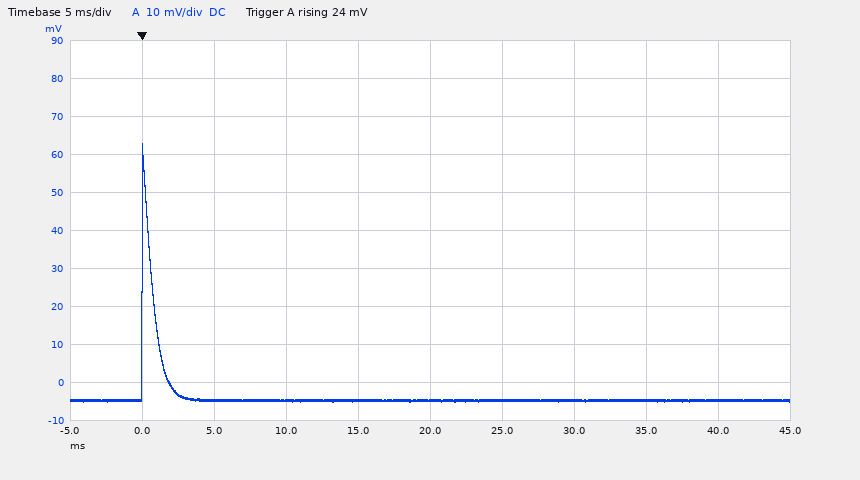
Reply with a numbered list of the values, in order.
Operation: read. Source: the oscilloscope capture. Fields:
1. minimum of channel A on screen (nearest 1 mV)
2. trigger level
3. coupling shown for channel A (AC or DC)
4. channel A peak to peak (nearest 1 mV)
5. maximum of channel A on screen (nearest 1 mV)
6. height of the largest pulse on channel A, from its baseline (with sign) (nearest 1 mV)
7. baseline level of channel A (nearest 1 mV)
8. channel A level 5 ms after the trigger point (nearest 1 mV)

1. -5 mV
2. 24 mV
3. DC
4. 68 mV
5. 63 mV
6. +68 mV
7. -5 mV
8. -5 mV
